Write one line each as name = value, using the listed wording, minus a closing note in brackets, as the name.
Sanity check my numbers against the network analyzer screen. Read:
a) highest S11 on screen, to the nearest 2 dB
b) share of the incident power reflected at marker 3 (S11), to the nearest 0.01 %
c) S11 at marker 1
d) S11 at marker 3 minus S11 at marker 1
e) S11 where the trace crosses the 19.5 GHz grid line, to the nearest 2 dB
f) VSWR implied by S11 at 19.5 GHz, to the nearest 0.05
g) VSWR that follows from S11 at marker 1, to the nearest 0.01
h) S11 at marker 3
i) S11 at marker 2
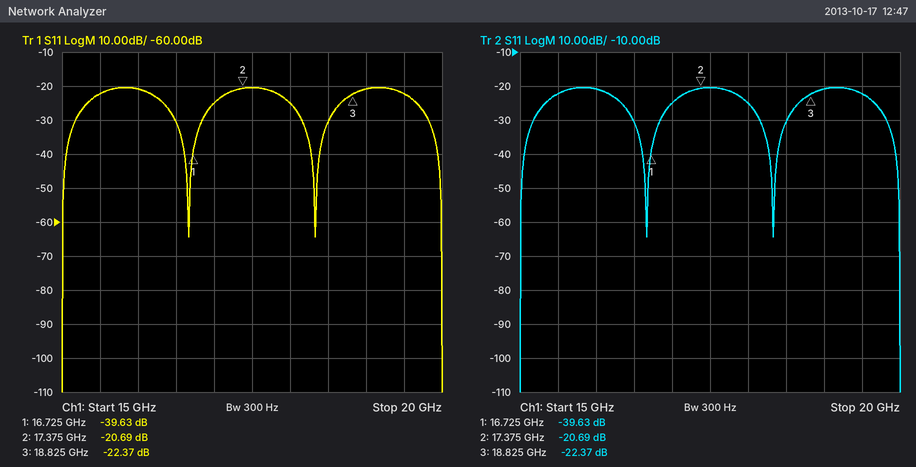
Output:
highest S11 on screen, to the nearest 2 dB = -20 dB
share of the incident power reflected at marker 3 (S11), to the nearest 0.01 % = 0.58 %
S11 at marker 1 = -39.63 dB
S11 at marker 3 minus S11 at marker 1 = 17.26 dB
S11 where the trace crosses the 19.5 GHz grid line, to the nearest 2 dB = -22 dB
VSWR implied by S11 at 19.5 GHz, to the nearest 0.05 = 1.15
VSWR that follows from S11 at marker 1, to the nearest 0.01 = 1.02
S11 at marker 3 = -22.37 dB
S11 at marker 2 = -20.69 dB
